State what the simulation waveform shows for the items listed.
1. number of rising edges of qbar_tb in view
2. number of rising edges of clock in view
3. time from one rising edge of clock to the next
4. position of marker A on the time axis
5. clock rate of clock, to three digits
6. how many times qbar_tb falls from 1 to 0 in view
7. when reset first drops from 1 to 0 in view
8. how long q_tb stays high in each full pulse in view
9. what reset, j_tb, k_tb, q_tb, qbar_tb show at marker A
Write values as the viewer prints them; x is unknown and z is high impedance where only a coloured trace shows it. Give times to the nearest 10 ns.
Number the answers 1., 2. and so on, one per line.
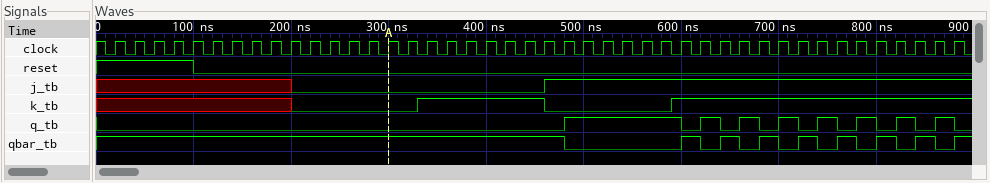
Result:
1. 8
2. 44
3. 20 ns
4. 300 ns
5. 50.0 MHz
6. 8
7. 100 ns
8. 120 ns, 20 ns, 20 ns, 20 ns, 20 ns, 20 ns, 20 ns, 20 ns
9. reset=0, j_tb=0, k_tb=0, q_tb=0, qbar_tb=1
